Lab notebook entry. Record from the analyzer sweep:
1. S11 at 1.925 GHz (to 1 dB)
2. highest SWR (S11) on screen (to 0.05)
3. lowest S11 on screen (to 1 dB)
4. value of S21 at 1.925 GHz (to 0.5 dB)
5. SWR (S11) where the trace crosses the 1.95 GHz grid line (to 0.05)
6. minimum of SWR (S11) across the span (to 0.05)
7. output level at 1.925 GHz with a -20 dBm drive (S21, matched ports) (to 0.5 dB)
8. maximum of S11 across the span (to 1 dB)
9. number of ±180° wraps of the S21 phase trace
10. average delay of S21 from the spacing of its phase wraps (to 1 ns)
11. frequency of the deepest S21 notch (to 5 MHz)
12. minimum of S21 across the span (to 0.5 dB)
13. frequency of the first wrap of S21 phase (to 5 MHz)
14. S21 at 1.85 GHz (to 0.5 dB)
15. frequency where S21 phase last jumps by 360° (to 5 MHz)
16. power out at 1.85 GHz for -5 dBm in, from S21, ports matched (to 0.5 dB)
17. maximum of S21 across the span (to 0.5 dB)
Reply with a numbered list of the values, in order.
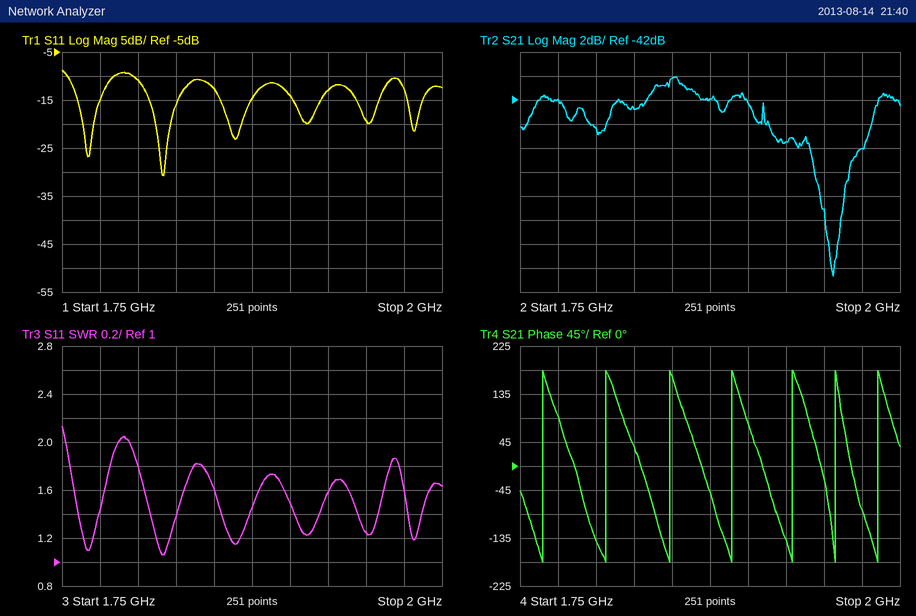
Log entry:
1. -13 dB
2. 2.15
3. -31 dB
4. -45.5 dB
5. 1.25
6. 1.05
7. -65.5 dBm
8. -9 dB
9. 7
10. 27 ns
11. 1.955 GHz
12. -56.5 dB
13. 1.765 GHz
14. -40.0 dB
15. 1.985 GHz
16. -45.0 dBm
17. -40.0 dB
